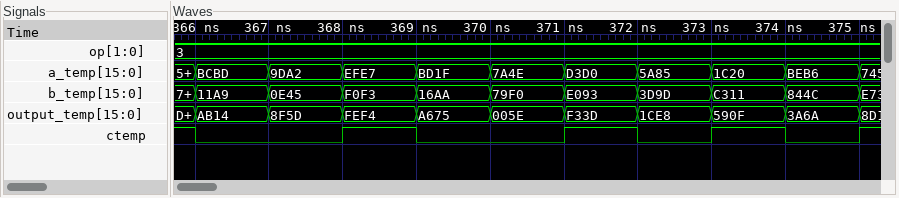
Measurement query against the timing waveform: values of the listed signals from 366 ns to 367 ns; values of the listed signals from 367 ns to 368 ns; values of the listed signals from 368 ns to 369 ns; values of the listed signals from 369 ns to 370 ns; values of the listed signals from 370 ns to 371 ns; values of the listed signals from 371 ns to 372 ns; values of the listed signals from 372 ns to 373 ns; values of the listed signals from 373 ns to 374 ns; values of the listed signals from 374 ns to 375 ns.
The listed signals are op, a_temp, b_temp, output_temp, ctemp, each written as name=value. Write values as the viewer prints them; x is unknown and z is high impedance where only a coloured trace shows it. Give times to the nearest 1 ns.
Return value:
op=3, a_temp=BCBD, b_temp=11A9, output_temp=AB14, ctemp=0
op=3, a_temp=9DA2, b_temp=0E45, output_temp=8F5D, ctemp=0
op=3, a_temp=EFE7, b_temp=F0F3, output_temp=FEF4, ctemp=1
op=3, a_temp=BD1F, b_temp=16AA, output_temp=A675, ctemp=0
op=3, a_temp=7A4E, b_temp=79F0, output_temp=005E, ctemp=0
op=3, a_temp=D3D0, b_temp=E093, output_temp=F33D, ctemp=1
op=3, a_temp=5A85, b_temp=3D9D, output_temp=1CE8, ctemp=0
op=3, a_temp=1C20, b_temp=C311, output_temp=590F, ctemp=1
op=3, a_temp=BEB6, b_temp=844C, output_temp=3A6A, ctemp=0
